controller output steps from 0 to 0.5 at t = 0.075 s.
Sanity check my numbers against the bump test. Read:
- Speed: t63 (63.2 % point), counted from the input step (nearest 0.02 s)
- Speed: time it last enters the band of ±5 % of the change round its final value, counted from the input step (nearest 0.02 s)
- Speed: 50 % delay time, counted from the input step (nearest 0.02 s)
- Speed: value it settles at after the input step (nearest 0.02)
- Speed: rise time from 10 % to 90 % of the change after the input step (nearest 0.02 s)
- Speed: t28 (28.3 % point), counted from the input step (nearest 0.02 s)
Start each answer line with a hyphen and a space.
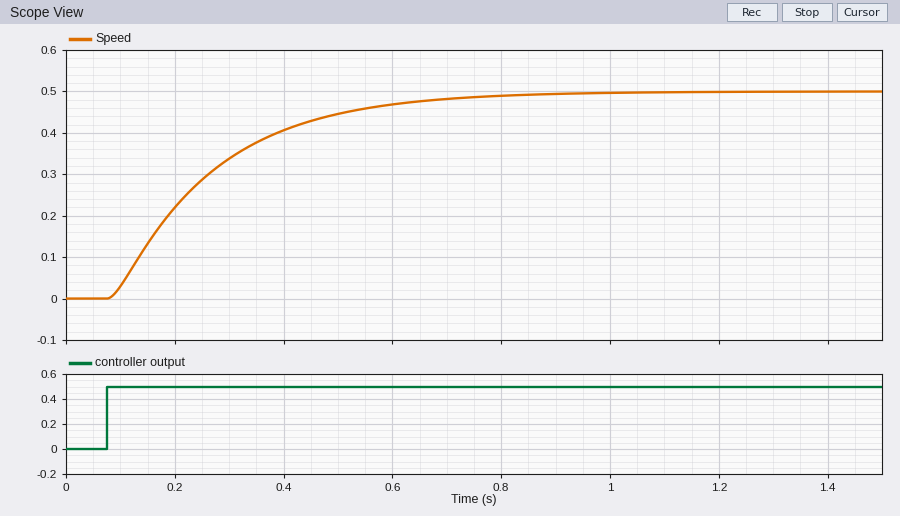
- 0.20 s
- 0.56 s
- 0.14 s
- 0.50
- 0.40 s
- 0.08 s
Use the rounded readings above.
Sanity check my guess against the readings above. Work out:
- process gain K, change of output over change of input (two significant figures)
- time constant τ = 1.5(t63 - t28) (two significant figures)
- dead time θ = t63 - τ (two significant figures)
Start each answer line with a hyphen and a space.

- 1.0
- 0.18 s
- 0.020 s
